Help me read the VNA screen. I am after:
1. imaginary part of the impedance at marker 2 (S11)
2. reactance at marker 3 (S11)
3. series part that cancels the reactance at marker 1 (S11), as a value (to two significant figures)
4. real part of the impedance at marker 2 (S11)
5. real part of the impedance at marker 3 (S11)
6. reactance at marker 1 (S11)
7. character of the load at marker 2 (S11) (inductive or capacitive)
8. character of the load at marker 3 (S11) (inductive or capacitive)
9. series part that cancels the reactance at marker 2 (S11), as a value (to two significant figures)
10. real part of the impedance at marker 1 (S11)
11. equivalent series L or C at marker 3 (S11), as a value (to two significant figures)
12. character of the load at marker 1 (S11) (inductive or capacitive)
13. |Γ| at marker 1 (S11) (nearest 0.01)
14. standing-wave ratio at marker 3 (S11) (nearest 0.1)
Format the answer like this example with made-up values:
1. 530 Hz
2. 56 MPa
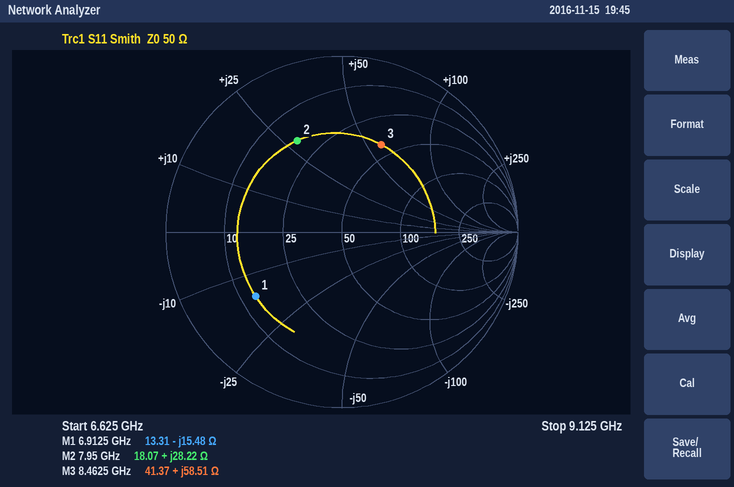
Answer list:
1. +28.22 Ω
2. +58.51 Ω
3. 360 pH
4. 18.07 Ω
5. 41.37 Ω
6. -15.48 Ω
7. inductive
8. inductive
9. 710 fF
10. 13.31 Ω
11. 1.1 nH
12. capacitive
13. 0.61
14. 3.4
